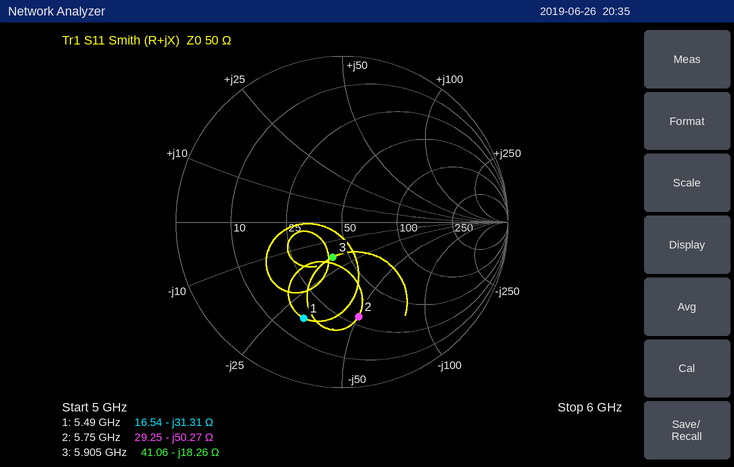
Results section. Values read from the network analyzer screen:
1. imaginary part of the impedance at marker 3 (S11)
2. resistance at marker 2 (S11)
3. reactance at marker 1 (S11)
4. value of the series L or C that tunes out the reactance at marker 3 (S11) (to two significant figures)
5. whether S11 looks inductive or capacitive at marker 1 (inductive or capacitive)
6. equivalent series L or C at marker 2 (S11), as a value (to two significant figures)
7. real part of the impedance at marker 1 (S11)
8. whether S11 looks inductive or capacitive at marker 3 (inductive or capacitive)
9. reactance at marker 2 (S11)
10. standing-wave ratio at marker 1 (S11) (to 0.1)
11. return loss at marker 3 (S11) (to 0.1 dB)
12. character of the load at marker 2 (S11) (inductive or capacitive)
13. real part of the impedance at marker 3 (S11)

-18.26 Ω
29.25 Ω
-31.31 Ω
490 pH
capacitive
550 fF
16.54 Ω
capacitive
-50.27 Ω
4.3
13.2 dB
capacitive
41.06 Ω
